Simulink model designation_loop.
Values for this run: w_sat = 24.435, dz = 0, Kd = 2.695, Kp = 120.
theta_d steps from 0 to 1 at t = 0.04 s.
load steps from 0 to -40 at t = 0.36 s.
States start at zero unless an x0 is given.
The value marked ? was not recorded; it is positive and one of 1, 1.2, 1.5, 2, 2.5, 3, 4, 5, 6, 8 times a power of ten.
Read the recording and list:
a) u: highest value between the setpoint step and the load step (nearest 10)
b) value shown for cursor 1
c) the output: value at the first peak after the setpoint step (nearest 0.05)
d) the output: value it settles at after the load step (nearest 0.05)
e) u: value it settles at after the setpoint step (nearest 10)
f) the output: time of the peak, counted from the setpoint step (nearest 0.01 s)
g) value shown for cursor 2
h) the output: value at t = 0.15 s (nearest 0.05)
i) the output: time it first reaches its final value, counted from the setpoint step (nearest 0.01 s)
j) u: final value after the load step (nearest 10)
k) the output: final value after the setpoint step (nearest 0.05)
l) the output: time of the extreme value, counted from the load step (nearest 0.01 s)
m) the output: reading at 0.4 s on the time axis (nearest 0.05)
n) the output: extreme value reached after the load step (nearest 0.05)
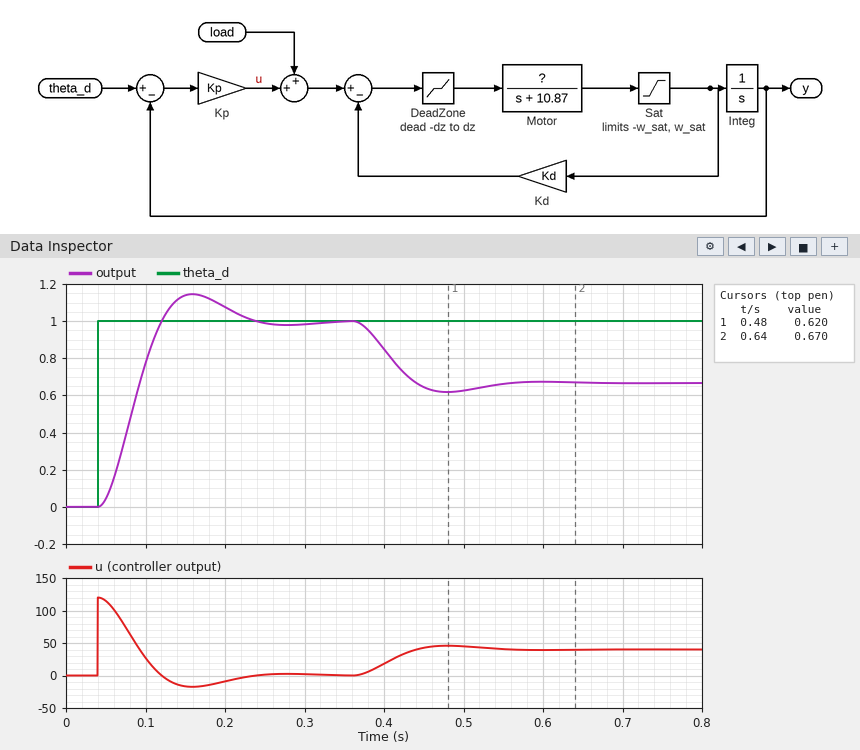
120
0.620
1.15
0.65
0
0.12 s
0.670
1.15
0.08 s
40
1.00
0.12 s
0.85
0.60
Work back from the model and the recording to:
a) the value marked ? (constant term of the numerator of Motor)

8
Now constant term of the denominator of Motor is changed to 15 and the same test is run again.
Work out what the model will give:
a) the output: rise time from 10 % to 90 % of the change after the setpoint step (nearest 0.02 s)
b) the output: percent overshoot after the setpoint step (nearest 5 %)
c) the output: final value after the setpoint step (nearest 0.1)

0.06 s
10 %
1.0
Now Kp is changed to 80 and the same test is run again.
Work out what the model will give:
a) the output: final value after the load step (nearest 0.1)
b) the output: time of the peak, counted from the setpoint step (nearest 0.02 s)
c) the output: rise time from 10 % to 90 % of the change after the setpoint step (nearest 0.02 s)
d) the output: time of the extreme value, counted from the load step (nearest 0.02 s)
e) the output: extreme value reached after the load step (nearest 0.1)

0.5
0.16 s
0.08 s
0.16 s
0.5
